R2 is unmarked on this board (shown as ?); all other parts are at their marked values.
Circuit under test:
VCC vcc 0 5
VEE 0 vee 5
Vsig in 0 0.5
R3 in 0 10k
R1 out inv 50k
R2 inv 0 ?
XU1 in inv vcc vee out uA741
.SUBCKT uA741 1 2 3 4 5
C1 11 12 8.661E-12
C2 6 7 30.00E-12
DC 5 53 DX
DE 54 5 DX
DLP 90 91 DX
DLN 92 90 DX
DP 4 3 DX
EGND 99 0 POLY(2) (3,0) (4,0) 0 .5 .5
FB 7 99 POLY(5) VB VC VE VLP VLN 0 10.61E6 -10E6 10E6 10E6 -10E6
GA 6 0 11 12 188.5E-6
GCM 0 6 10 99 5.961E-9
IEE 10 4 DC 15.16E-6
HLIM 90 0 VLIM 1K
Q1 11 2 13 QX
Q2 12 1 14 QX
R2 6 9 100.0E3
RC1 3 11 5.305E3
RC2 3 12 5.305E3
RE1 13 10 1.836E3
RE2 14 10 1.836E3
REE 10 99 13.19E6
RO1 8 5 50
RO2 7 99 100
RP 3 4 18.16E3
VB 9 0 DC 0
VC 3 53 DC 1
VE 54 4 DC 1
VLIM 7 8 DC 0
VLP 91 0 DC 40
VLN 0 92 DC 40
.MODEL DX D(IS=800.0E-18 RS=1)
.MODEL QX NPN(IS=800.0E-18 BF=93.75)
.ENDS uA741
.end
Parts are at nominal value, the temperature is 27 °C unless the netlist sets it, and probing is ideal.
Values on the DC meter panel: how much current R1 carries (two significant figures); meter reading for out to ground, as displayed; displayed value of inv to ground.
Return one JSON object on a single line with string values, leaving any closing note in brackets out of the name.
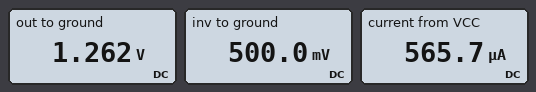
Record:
{"how much current R1 carries": "15 µA", "meter reading for out to ground, as displayed": "1.262 V", "displayed value of inv to ground": "500.0 mV"}
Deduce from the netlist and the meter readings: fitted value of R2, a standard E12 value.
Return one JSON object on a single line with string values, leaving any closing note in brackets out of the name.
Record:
{"fitted value of R2, a standard E12 value": "33 kΩ"}
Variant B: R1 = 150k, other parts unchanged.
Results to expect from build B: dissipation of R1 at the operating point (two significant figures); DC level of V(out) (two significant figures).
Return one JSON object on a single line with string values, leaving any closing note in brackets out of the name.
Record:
{"dissipation of R1 at the operating point": "35 µW", "DC level of V(out)": "2.8 V"}
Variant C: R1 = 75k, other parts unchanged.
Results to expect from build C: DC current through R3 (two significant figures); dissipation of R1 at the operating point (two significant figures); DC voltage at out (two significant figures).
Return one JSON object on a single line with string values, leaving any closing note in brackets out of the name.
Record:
{"DC current through R3": "50 µA", "dissipation of R1 at the operating point": "17 µW", "DC voltage at out": "1.6 V"}
